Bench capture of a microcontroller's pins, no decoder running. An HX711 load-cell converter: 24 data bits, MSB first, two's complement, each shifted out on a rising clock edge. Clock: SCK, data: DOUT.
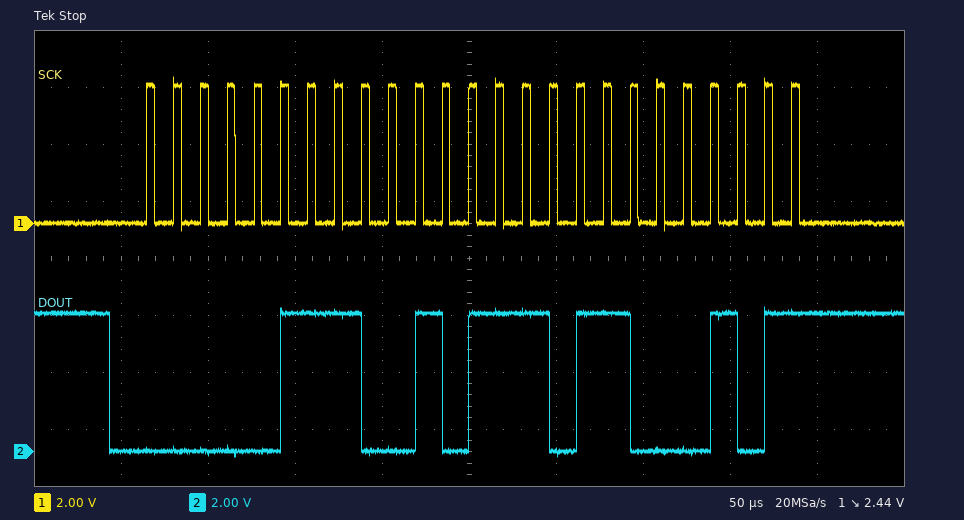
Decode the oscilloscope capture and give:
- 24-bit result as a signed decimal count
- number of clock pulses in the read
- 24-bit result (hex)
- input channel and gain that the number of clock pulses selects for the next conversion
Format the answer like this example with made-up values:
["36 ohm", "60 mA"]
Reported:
["470725", "25", "0x072EC5", "channel A, gain 128"]
